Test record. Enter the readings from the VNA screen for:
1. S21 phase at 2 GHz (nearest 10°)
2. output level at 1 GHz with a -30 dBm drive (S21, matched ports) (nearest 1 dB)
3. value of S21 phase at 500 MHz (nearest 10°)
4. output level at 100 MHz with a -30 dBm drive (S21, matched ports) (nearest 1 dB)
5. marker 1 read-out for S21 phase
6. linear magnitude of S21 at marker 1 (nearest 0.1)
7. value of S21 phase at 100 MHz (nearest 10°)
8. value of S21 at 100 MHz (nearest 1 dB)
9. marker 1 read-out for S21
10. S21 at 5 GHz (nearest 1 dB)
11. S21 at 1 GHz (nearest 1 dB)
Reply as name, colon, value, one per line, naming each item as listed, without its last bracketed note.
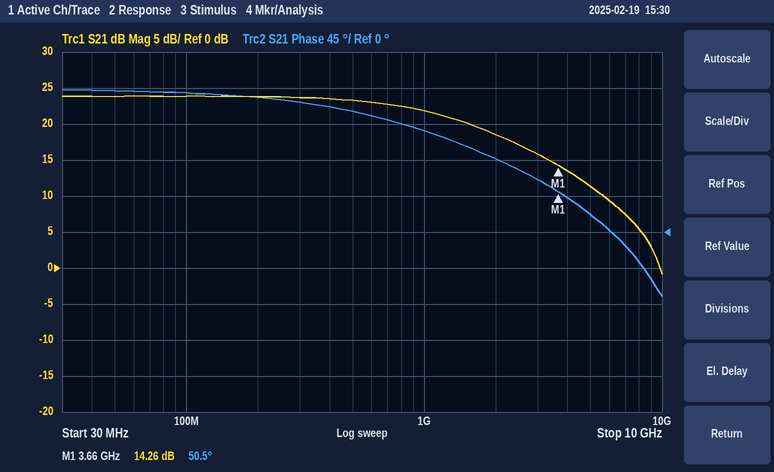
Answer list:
S21 phase at 2 GHz: 90°
output level at 1 GHz with a -30 dBm drive (S21, matched ports): -8 dBm
value of S21 phase at 500 MHz: 150°
output level at 100 MHz with a -30 dBm drive (S21, matched ports): -6 dBm
marker 1 read-out for S21 phase: 50.5°
linear magnitude of S21 at marker 1: 5.2
value of S21 phase at 100 MHz: 170°
value of S21 at 100 MHz: 24 dB
marker 1 read-out for S21: 14.26 dB
S21 at 5 GHz: 11 dB
S21 at 1 GHz: 22 dB
